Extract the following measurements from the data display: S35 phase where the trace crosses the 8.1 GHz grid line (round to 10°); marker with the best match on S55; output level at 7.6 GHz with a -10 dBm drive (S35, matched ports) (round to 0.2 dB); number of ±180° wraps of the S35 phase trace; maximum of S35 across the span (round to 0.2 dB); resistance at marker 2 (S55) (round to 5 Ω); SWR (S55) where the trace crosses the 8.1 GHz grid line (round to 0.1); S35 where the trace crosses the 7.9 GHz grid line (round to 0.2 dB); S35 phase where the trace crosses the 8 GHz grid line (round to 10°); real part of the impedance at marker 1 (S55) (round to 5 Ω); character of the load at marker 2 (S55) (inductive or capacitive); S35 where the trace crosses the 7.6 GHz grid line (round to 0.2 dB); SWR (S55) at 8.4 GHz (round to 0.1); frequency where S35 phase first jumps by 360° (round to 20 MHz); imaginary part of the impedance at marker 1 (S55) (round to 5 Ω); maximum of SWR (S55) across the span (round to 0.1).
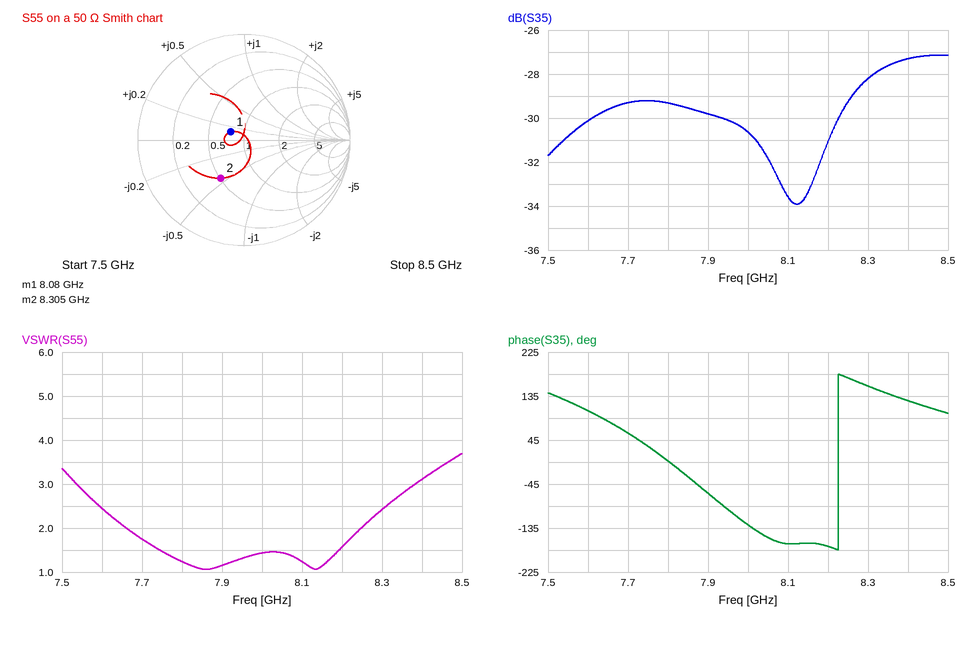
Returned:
-170°
marker 1
-40.2 dBm
1
-27.2 dB
25 Ω
1.2
-29.8 dB
-130°
40 Ω
capacitive
-30.2 dB
3.1
8.22 GHz
+5 Ω
3.7
